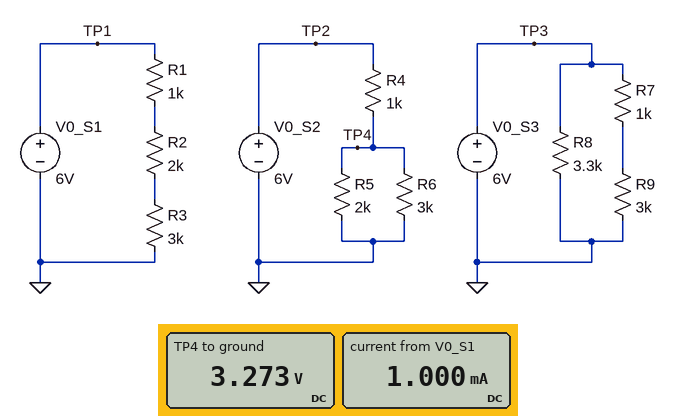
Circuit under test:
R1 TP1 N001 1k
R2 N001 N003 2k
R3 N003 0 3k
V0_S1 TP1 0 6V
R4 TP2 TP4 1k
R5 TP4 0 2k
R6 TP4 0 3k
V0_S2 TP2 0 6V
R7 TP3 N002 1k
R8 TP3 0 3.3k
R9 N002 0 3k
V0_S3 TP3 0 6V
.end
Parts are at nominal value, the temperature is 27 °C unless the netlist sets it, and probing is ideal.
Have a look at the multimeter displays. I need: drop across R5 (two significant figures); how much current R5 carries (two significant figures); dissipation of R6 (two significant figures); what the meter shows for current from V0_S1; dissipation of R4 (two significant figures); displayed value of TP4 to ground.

3.3 V
1.6 mA
3.6 mW
1.000 mA
7.4 mW
3.273 V
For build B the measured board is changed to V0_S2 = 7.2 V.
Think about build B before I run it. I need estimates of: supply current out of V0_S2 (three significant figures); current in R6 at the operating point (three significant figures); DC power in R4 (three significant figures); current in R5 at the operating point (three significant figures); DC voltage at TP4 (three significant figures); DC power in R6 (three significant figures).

3.27 mA
1.31 mA
10.7 mW
1.96 mA
3.93 V
5.14 mW
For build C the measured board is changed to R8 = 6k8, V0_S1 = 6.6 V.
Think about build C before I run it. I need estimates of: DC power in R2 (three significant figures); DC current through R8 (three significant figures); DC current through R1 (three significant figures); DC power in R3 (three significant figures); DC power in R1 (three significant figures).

2.42 mW
882 µA
1.10 mA
3.63 mW
1.21 mW
